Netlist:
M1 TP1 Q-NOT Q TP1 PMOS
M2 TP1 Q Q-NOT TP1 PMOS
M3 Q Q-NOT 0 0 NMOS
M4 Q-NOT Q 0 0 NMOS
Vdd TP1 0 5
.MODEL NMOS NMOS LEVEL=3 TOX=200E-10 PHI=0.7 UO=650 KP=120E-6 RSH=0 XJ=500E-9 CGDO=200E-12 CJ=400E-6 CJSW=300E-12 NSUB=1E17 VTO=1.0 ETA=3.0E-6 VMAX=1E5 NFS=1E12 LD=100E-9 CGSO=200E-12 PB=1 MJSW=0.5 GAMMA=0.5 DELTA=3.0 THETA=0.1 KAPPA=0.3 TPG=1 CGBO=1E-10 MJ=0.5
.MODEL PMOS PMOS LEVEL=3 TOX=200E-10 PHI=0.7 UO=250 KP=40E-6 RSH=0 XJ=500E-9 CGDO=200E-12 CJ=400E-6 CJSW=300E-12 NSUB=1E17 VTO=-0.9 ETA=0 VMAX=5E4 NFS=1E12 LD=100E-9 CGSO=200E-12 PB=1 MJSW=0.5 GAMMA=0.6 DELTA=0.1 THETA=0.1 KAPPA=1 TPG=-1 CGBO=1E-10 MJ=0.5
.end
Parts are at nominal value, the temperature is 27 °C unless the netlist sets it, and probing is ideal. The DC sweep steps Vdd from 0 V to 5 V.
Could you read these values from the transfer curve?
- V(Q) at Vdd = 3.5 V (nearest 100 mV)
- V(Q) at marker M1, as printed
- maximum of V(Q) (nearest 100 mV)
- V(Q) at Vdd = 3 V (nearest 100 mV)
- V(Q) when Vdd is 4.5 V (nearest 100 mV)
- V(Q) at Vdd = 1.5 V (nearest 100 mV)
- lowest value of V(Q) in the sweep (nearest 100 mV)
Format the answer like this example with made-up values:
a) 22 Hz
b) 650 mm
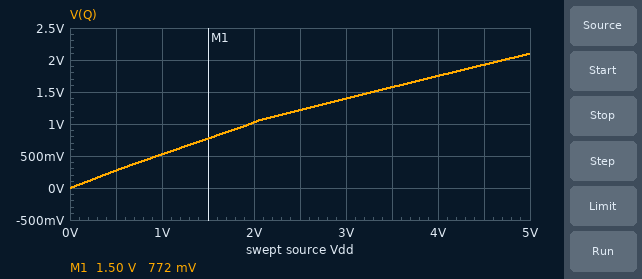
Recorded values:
a) 1.6 V
b) 772 mV
c) 2.1 V
d) 1.4 V
e) 1.9 V
f) 800 mV
g) 0 V
